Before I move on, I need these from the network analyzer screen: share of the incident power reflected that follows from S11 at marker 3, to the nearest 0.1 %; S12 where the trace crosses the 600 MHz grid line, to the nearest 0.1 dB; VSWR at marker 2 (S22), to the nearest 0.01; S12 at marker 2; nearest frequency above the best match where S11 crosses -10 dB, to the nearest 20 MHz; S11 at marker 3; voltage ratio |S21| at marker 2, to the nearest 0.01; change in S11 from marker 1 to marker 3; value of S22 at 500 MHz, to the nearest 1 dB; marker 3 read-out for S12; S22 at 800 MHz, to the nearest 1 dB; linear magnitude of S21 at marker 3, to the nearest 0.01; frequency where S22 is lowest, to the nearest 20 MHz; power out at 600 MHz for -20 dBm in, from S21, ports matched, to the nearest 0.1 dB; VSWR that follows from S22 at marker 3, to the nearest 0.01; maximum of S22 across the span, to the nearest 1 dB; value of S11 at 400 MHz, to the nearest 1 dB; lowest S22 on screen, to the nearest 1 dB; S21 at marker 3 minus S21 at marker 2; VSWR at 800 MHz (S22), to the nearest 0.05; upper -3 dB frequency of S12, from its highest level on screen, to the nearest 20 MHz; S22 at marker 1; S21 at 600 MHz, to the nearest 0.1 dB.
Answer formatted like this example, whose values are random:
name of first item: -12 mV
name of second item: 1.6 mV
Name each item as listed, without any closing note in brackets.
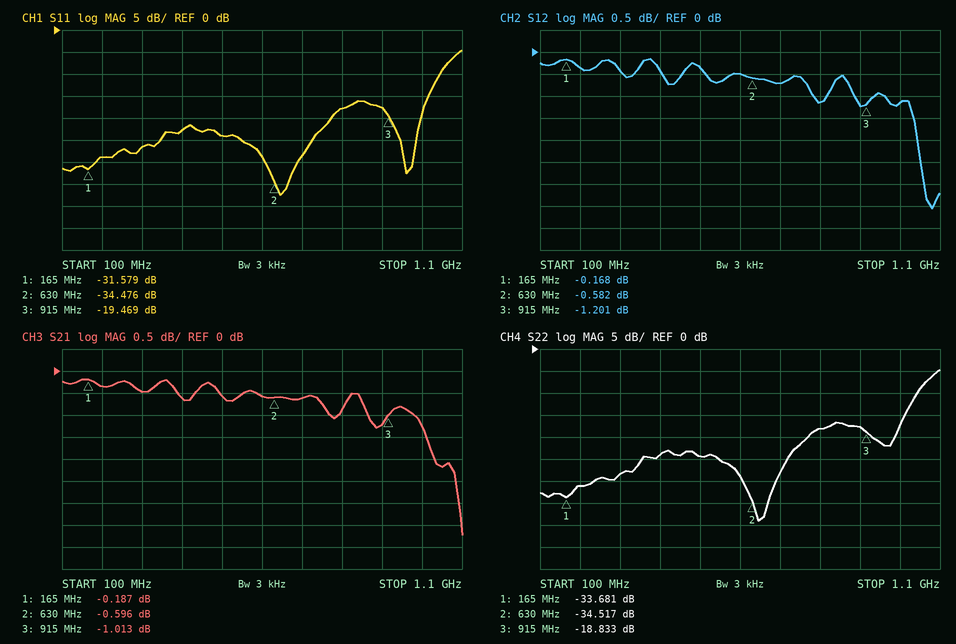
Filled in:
share of the incident power reflected that follows from S11 at marker 3, to the nearest 0.1 %: 1.1 %
S12 where the trace crosses the 600 MHz grid line, to the nearest 0.1 dB: -0.5 dB
VSWR at marker 2 (S22), to the nearest 0.01: 1.04
S12 at marker 2: -0.582 dB
nearest frequency above the best match where S11 crosses -10 dB, to the nearest 20 MHz: 1.04 GHz
S11 at marker 3: -19.469 dB
voltage ratio |S21| at marker 2, to the nearest 0.01: 0.93
change in S11 from marker 1 to marker 3: 12.110 dB
value of S22 at 500 MHz, to the nearest 1 dB: -24 dB
marker 3 read-out for S12: -1.201 dB
S22 at 800 MHz, to the nearest 1 dB: -18 dB
linear magnitude of S21 at marker 3, to the nearest 0.01: 0.89
frequency where S22 is lowest, to the nearest 20 MHz: 640 MHz
power out at 600 MHz for -20 dBm in, from S21, ports matched, to the nearest 0.1 dB: -20.6 dBm
VSWR that follows from S22 at marker 3, to the nearest 0.01: 1.26
maximum of S22 across the span, to the nearest 1 dB: -5 dB
value of S11 at 400 MHz, to the nearest 1 dB: -23 dB
lowest S22 on screen, to the nearest 1 dB: -39 dB
S21 at marker 3 minus S21 at marker 2: -0.417 dB
VSWR at 800 MHz (S22), to the nearest 0.05: 1.30
upper -3 dB frequency of S12, from its highest level on screen, to the nearest 20 MHz: 1.06 GHz
S22 at marker 1: -33.681 dB
S21 at 600 MHz, to the nearest 0.1 dB: -0.6 dB
